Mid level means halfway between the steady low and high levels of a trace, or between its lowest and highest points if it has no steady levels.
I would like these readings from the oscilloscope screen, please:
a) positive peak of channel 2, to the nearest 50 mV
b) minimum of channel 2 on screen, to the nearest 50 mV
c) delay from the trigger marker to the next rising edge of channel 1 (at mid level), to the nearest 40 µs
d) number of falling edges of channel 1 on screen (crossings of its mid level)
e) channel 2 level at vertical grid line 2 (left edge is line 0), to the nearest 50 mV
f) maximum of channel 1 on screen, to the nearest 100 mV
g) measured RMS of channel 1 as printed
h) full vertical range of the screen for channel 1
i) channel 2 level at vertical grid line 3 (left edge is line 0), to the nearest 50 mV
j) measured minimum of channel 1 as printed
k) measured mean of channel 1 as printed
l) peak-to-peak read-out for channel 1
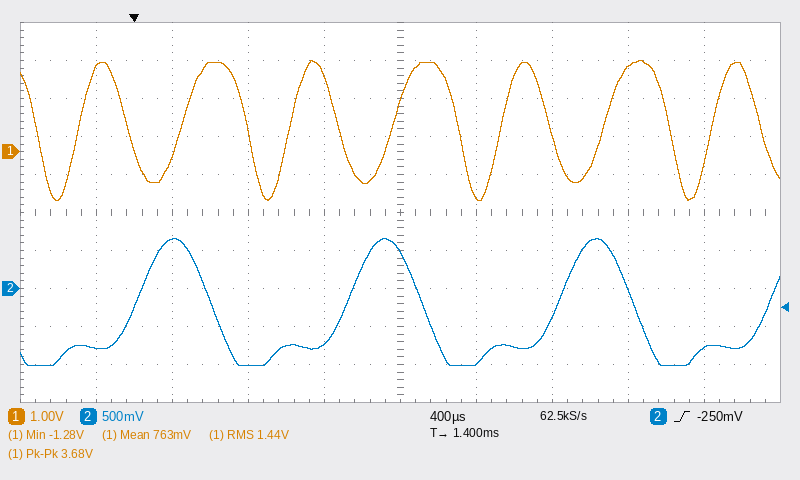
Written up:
650 mV
-1.00 V
240 µs
8
650 mV
2.4 V
1.44 V
10 V
-1.00 V
-1.28 V
763 mV
3.68 V
